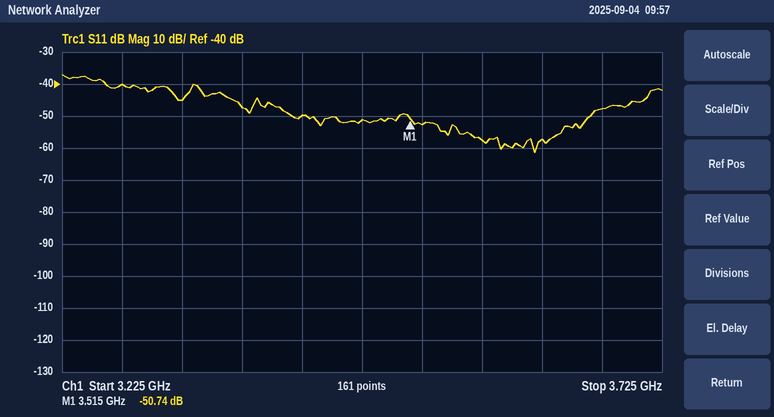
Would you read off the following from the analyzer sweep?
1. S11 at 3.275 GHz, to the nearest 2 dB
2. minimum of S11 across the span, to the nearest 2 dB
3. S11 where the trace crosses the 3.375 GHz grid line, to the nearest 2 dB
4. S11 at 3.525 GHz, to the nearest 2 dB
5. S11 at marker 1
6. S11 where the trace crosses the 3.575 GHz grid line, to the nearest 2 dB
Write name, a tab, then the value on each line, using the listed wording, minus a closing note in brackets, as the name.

S11 at 3.275 GHz, to the nearest 2 dB	-40 dB
minimum of S11 across the span, to the nearest 2 dB	-62 dB
S11 where the trace crosses the 3.375 GHz grid line, to the nearest 2 dB	-48 dB
S11 at 3.525 GHz, to the nearest 2 dB	-52 dB
S11 at marker 1	-50.74 dB
S11 where the trace crosses the 3.575 GHz grid line, to the nearest 2 dB	-58 dB
